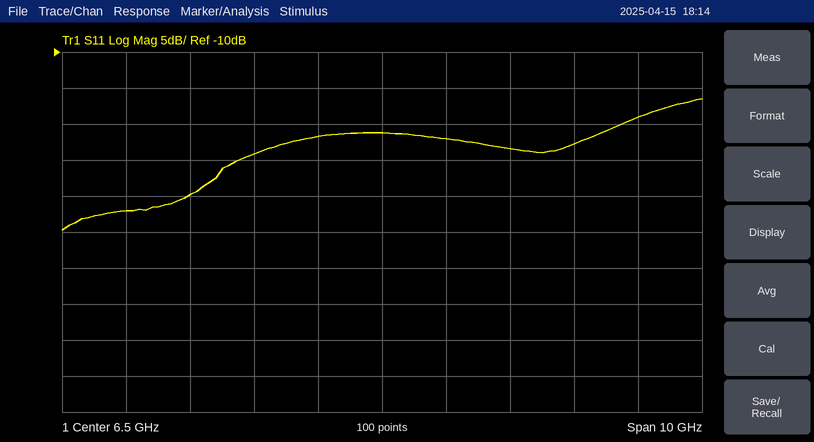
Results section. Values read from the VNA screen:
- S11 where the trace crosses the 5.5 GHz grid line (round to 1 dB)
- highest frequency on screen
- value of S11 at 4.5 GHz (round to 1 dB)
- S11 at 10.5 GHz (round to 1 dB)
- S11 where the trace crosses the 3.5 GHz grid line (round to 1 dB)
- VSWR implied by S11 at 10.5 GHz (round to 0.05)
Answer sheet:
-22 dB
11.5 GHz
-24 dB
-19 dB
-30 dB
1.25
